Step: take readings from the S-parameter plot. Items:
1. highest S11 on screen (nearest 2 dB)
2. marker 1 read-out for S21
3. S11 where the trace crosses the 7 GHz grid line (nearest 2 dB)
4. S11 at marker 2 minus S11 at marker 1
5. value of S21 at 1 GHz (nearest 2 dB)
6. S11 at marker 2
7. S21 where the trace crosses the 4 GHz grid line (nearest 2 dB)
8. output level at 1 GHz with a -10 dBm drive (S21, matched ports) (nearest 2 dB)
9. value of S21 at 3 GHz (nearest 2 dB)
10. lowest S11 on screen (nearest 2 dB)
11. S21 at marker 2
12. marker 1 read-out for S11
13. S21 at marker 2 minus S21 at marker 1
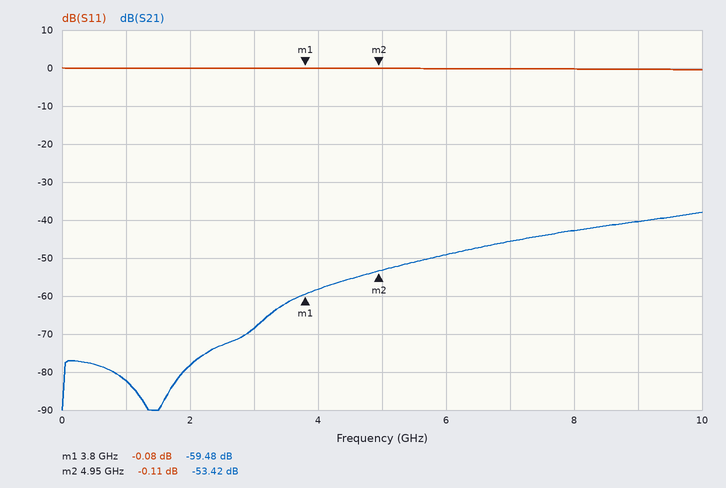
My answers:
0 dB
-59.48 dB
0 dB
-0.03 dB
-82 dB
-0.11 dB
-58 dB
-92 dBm
-68 dB
0 dB
-53.42 dB
-0.08 dB
6.06 dB
